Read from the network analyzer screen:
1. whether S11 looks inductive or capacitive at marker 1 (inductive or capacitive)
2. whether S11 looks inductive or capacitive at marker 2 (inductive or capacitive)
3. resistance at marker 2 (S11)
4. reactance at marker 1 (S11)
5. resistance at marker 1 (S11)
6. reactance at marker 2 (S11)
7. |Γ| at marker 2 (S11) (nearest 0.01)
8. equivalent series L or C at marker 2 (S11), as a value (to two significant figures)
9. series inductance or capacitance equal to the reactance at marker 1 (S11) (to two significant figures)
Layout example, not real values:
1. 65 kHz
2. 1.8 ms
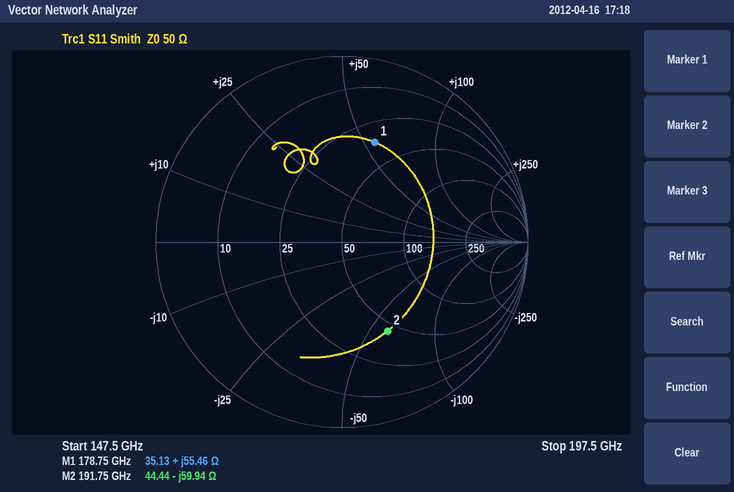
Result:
1. inductive
2. capacitive
3. 44.44 Ω
4. +55.46 Ω
5. 35.13 Ω
6. -59.94 Ω
7. 0.54
8. 14 fF
9. 49 pH
